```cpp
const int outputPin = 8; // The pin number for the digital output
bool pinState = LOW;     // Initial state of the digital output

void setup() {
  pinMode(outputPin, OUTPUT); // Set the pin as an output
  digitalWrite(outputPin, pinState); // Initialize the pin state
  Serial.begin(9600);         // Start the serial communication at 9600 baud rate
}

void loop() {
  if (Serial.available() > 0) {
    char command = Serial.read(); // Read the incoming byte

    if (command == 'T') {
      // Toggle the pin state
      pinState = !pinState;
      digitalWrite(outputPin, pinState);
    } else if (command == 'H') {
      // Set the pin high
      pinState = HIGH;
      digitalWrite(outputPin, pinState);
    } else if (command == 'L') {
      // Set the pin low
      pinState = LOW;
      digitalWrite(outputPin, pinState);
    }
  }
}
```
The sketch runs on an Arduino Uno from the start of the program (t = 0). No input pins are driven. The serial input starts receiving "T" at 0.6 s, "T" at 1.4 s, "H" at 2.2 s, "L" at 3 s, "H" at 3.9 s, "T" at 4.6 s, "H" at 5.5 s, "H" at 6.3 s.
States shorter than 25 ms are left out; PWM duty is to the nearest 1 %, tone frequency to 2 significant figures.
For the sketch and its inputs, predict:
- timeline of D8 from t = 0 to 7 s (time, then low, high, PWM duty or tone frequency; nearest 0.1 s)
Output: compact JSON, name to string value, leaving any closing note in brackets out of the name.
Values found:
{"timeline of D8 from t = 0 to 7 s": "0 s low; 0.6 s high; 1.4 s low; 2.2 s high; 3 s low; 3.9 s high; 4.6 s low; 5.5 s high"}
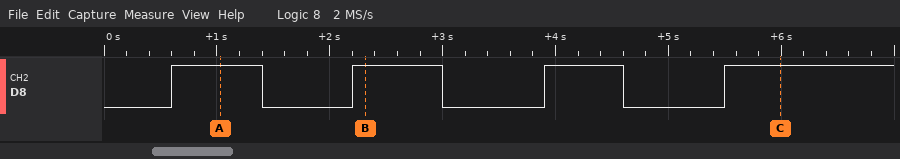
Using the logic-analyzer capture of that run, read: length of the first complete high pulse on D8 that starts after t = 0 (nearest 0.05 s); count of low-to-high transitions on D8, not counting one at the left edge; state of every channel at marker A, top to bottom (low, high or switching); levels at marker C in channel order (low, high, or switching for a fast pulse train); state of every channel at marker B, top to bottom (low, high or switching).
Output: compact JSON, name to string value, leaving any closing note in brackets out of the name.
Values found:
{"length of the first complete high pulse on D8 that starts after t = 0": "0.80 s", "count of low-to-high transitions on D8, not counting one at the left edge": "4", "state of every channel at marker A, top to bottom": "D8 high", "levels at marker C in channel order": "D8 high", "state of every channel at marker B, top to bottom": "D8 high"}
